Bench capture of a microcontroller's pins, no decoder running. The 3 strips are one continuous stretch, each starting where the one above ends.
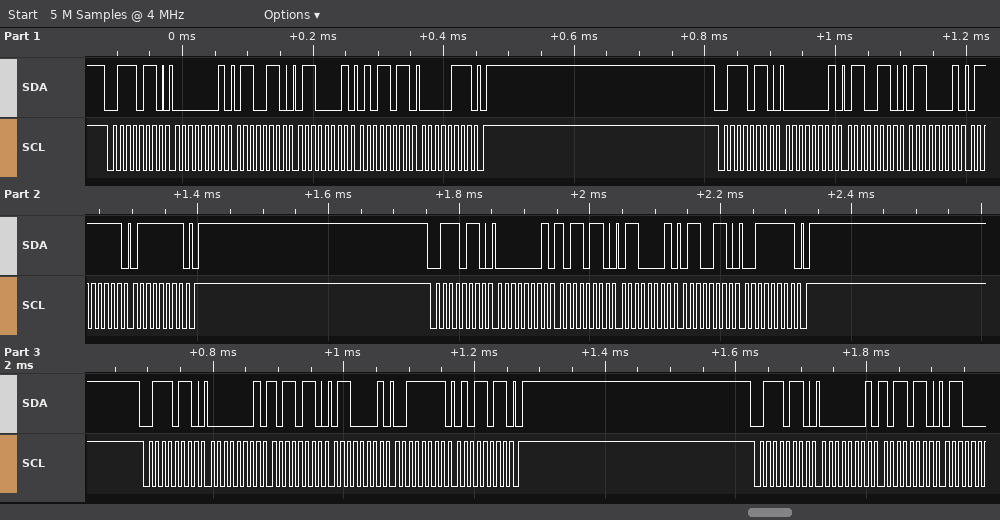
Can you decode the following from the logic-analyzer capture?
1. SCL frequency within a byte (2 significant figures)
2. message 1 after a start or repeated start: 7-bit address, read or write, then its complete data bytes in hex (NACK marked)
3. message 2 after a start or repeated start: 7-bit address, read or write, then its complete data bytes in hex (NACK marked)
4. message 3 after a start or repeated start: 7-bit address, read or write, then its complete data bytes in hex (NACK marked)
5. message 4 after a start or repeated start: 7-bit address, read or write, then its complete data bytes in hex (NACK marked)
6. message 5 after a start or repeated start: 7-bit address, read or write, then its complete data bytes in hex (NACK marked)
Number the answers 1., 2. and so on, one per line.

1. 100 kHz
2. 0x3B write: 01 66 61 5B 07
3. 0x3B write: 01 66 61 7F 7F
4. 0x3B write: 01 B6 61 66 3F
5. 0x3B write: 01 B6 61 3F 5B
6. 0x3B write: 01 B6
